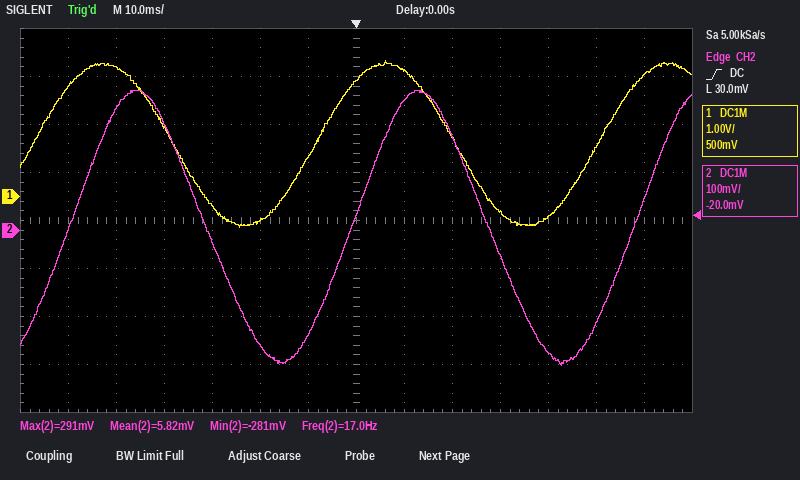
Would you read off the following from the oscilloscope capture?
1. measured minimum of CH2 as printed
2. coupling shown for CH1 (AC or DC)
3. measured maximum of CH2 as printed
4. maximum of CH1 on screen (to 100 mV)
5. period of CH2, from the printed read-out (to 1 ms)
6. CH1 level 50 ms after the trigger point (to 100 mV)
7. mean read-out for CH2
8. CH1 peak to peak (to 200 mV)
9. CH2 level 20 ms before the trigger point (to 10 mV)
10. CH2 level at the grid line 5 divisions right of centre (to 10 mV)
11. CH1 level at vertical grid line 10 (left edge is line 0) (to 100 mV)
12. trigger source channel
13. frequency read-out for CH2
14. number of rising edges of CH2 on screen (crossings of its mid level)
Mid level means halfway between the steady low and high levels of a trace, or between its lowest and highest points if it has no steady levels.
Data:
-281 mV
DC
291 mV
2.8 V
59 ms
1.0 V
5.82 mV
3.4 V
-240 mV
-190 mV
-300 mV
CH2
17.0 Hz
3
